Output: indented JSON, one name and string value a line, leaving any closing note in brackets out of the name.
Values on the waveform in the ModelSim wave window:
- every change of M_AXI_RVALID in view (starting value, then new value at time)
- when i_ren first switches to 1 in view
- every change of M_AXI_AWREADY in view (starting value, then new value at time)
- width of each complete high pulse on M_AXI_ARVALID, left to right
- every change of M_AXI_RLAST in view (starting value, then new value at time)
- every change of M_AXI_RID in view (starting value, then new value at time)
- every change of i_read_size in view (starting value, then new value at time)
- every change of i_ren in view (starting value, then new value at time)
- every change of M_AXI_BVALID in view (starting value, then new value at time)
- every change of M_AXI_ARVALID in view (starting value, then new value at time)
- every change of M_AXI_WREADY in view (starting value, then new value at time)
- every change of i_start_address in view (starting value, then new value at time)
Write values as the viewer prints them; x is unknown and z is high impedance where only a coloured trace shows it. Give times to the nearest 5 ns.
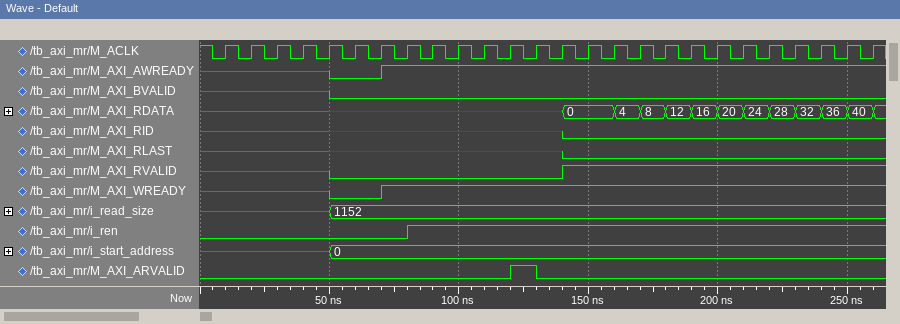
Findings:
{
  "every change of M_AXI_RVALID in view": "z, 0 at 50 ns, 1 at 140 ns",
  "when i_ren first switches to 1 in view": "80 ns",
  "every change of M_AXI_AWREADY in view": "z, 0 at 50 ns, 1 at 70 ns",
  "width of each complete high pulse on M_AXI_ARVALID, left to right": "10 ns",
  "every change of M_AXI_RLAST in view": "z, x at 50 ns, 0 at 140 ns",
  "every change of M_AXI_RID in view": "z, x at 50 ns, 0 at 140 ns",
  "every change of i_read_size in view": "z, 1152 at 50 ns",
  "every change of i_ren in view": "0, 1 at 80 ns",
  "every change of M_AXI_BVALID in view": "z, 0 at 50 ns",
  "every change of M_AXI_ARVALID in view": "0, 1 at 120 ns, 0 at 130 ns",
  "every change of M_AXI_WREADY in view": "z, 0 at 50 ns, 1 at 70 ns",
  "every change of i_start_address in view": "z, 0 at 50 ns"
}
